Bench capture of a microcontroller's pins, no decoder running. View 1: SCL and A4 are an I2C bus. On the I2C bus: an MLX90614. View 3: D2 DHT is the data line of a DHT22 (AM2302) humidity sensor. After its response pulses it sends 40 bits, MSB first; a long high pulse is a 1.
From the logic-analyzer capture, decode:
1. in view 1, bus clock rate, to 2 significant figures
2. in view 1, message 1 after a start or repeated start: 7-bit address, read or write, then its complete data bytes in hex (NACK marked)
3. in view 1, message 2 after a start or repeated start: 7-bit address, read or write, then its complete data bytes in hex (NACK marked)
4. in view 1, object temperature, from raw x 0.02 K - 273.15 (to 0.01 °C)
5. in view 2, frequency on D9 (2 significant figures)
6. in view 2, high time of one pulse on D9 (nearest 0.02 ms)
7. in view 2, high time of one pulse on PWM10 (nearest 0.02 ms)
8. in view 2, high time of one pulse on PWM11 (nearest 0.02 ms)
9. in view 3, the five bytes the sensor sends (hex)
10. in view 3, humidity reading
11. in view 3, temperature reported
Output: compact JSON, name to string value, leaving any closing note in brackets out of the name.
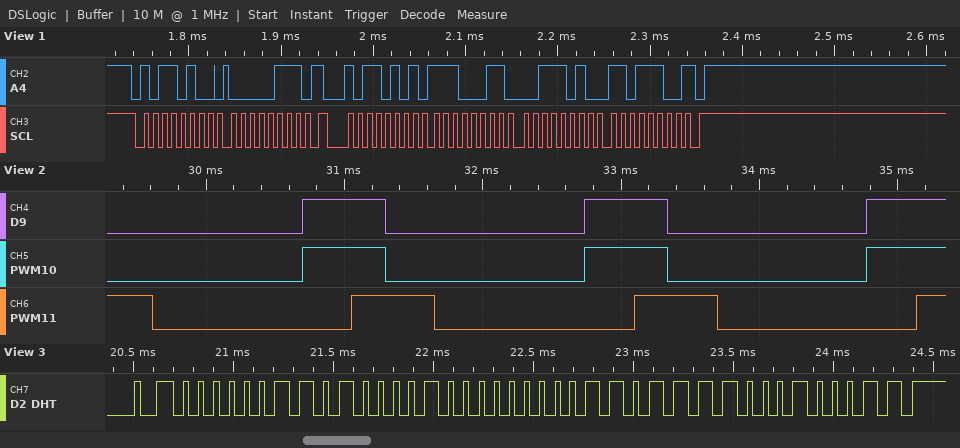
{"in view 1, bus clock rate, to 2 significant figures": "100 kHz", "in view 1, message 1 after a start or repeated start: 7-bit address, read or write, then its complete data bytes in hex": "0x5A write: 07", "in view 1, message 2 after a start or repeated start: 7-bit address, read or write, then its complete data bytes in hex": "0x5A read: E3 3A DC NACK", "in view 1, object temperature, from raw x 0.02 K - 273.15": "28.35 °C", "in view 2, frequency on D9": "490 Hz", "in view 2, high time of one pulse on D9": "0.60 ms", "in view 2, high time of one pulse on PWM10": "0.60 ms", "in view 2, high time of one pulse on PWM11": "0.60 ms", "in view 3, the five bytes the sensor sends": "03 42 00 DE 23", "in view 3, humidity reading": "83.4 %", "in view 3, temperature reported": "22.2 °C"}
